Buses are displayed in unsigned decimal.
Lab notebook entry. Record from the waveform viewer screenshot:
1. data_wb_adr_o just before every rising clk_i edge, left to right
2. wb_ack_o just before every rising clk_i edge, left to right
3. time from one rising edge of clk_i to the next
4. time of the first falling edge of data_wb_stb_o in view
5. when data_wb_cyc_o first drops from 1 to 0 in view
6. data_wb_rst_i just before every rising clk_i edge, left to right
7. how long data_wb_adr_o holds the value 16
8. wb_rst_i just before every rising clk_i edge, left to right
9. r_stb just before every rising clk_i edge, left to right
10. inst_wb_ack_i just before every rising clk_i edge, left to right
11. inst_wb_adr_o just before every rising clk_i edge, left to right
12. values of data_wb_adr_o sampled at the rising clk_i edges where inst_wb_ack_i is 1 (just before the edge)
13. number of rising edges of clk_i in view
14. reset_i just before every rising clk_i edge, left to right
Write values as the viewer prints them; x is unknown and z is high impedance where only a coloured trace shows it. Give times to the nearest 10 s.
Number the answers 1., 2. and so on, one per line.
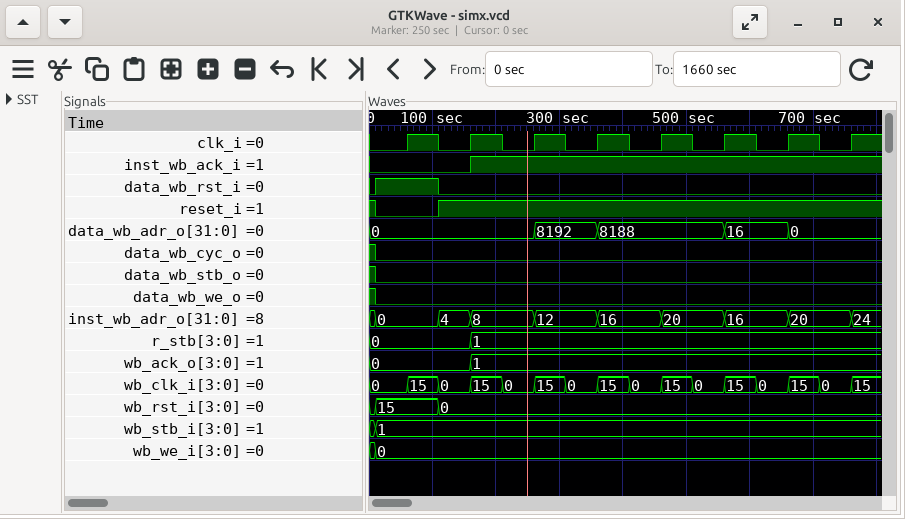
1. 0, 0, 0, 8192, 8188, 8188, 16, 0
2. 0, 0, 1, 1, 1, 1, 1, 1
3. 100 s
4. 10 s
5. 10 s
6. 1 0 0 0 0 0 0 0
7. 100 s
8. 15, 0, 0, 0, 0, 0, 0, 0
9. 0, 0, 1, 1, 1, 1, 1, 1
10. 0 0 1 1 1 1 1 1
11. 0, 4, 8, 12, 16, 20, 16, 20
12. 0, 8192, 8188, 8188, 16, 0
13. 8
14. 0 1 1 1 1 1 1 1
